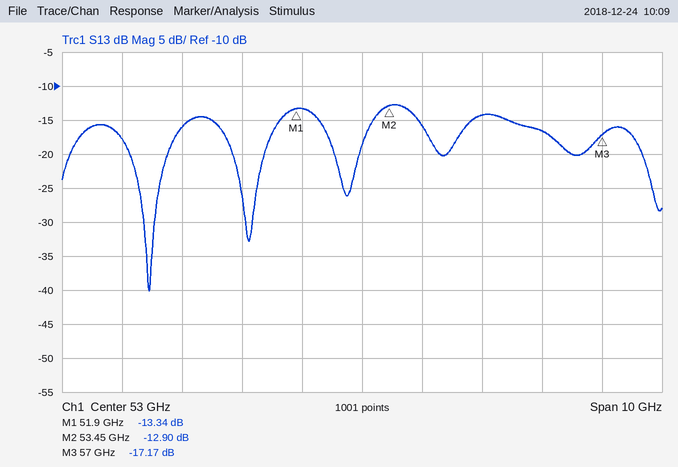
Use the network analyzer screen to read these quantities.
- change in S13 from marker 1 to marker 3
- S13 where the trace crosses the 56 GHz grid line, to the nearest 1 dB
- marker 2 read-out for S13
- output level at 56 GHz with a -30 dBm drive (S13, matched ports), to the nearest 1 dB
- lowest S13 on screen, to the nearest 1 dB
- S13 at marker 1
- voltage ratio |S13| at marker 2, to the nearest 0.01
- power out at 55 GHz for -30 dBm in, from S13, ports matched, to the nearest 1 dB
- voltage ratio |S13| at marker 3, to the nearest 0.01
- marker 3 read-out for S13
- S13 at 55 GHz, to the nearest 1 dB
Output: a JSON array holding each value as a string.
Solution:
["-3.83 dB", "-17 dB", "-12.90 dB", "-47 dBm", "-40 dB", "-13.34 dB", "0.23", "-44 dBm", "0.14", "-17.17 dB", "-14 dB"]
